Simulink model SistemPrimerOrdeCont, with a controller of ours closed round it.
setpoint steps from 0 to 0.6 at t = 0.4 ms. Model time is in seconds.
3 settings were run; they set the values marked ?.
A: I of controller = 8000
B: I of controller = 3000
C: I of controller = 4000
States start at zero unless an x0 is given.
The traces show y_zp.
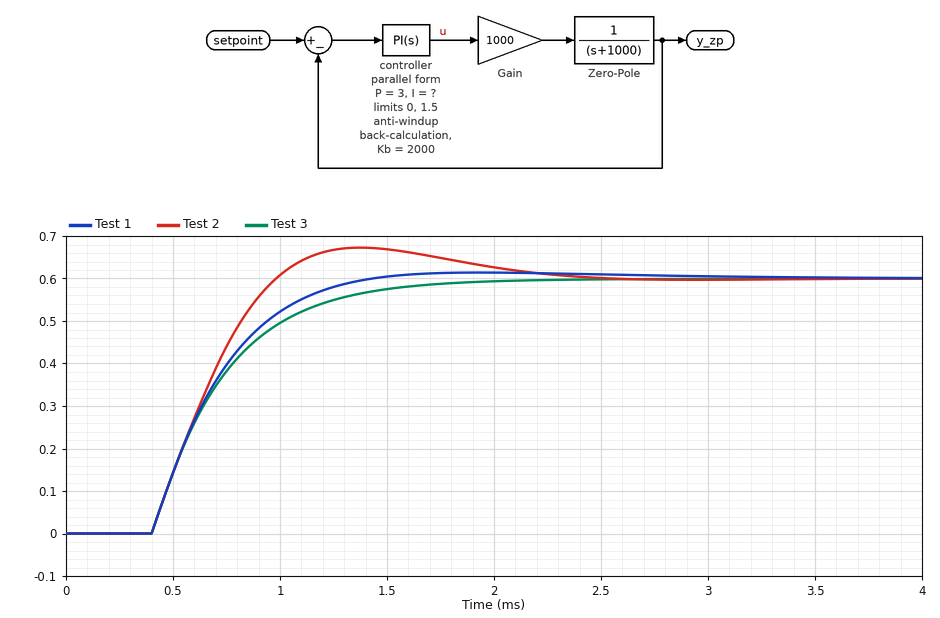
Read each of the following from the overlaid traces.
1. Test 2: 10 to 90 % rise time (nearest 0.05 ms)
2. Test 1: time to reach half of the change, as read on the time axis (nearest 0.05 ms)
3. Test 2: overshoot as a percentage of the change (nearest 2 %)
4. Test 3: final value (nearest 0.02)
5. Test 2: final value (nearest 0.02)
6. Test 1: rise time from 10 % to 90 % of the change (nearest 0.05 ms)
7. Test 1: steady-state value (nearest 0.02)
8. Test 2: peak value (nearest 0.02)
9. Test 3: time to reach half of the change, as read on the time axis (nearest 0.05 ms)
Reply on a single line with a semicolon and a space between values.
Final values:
0.45 ms; 0.65 ms; 12 %; 0.60; 0.60; 0.60 ms; 0.60; 0.68; 0.65 ms
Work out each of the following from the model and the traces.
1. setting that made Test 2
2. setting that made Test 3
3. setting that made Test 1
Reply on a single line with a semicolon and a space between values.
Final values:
A; B; C
